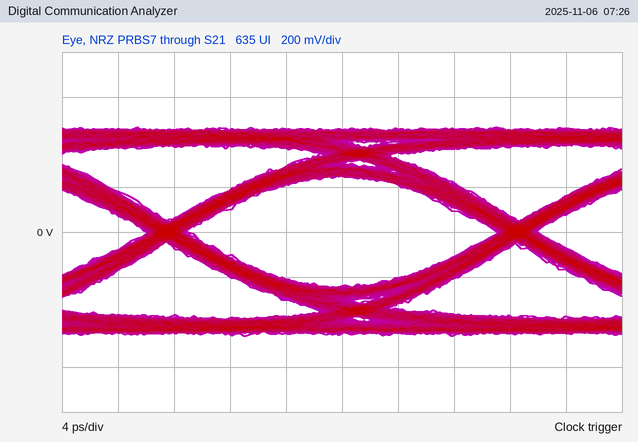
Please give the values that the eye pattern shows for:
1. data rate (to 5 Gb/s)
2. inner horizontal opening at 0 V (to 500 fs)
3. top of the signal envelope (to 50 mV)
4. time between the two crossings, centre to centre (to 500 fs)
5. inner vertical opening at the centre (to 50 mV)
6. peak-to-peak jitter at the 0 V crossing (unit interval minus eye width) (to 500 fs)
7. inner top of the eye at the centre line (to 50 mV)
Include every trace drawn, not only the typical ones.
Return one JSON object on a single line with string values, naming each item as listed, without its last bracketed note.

{"data rate": "40 Gb/s", "inner horizontal opening at 0 V": "22.0 ps", "top of the signal envelope": "450 mV", "time between the two crossings, centre to centre": "25.0 ps", "inner vertical opening at the centre": "500 mV", "peak-to-peak jitter at the 0 V crossing (unit interval minus eye width)": "3.0 ps", "inner top of the eye at the centre line": "250 mV"}
